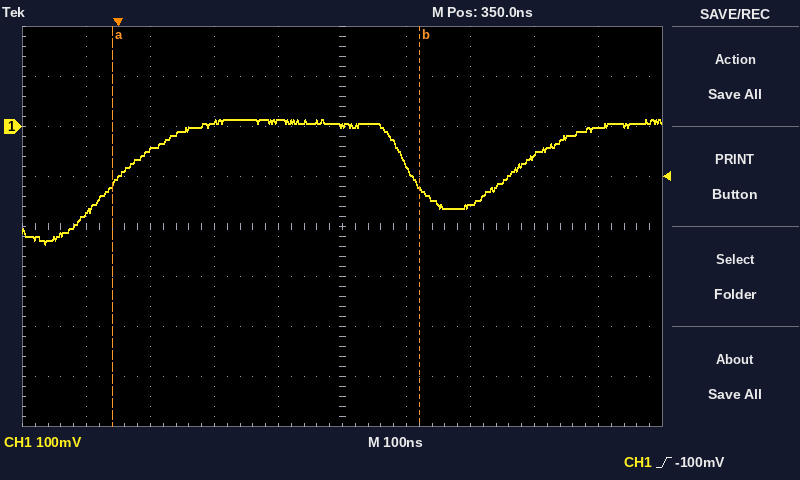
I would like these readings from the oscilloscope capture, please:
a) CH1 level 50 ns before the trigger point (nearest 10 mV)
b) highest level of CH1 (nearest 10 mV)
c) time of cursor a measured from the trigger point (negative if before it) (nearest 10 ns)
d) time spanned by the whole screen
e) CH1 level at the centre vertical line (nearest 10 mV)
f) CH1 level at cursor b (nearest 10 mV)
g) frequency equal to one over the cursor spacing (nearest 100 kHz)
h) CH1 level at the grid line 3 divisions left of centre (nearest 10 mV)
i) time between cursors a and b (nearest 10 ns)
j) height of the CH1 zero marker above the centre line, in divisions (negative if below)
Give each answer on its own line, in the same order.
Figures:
-170 mV
10 mV
-10 ns
1 µs
0 mV
-120 mV
2.1 MHz
-50 mV
480 ns
+2.0 div
